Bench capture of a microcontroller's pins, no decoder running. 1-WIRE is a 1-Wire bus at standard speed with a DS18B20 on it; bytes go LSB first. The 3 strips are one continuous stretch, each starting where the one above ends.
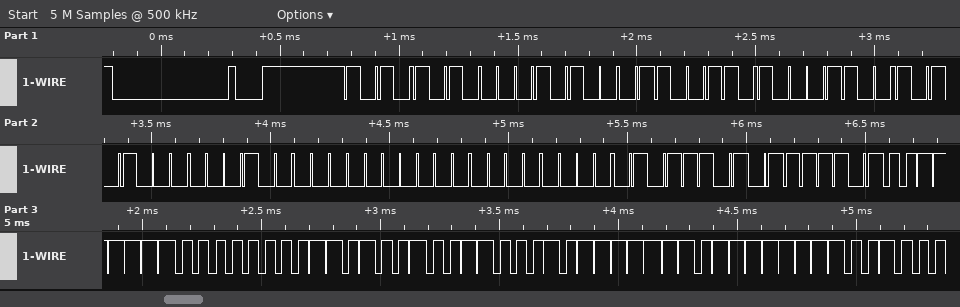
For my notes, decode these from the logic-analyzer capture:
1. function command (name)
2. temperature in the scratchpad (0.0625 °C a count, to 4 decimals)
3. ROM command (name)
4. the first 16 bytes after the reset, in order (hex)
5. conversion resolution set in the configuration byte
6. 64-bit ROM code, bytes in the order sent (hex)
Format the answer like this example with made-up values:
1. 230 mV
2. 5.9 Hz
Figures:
1. Read Scratchpad
2. 15.7500 °C
3. Match ROM
4. 55 28 66 31 15 08 00 00 BA BE FC 00 4B 46 7F FF
5. 12 bits
6. 28 66 31 15 08 00 00 BA
